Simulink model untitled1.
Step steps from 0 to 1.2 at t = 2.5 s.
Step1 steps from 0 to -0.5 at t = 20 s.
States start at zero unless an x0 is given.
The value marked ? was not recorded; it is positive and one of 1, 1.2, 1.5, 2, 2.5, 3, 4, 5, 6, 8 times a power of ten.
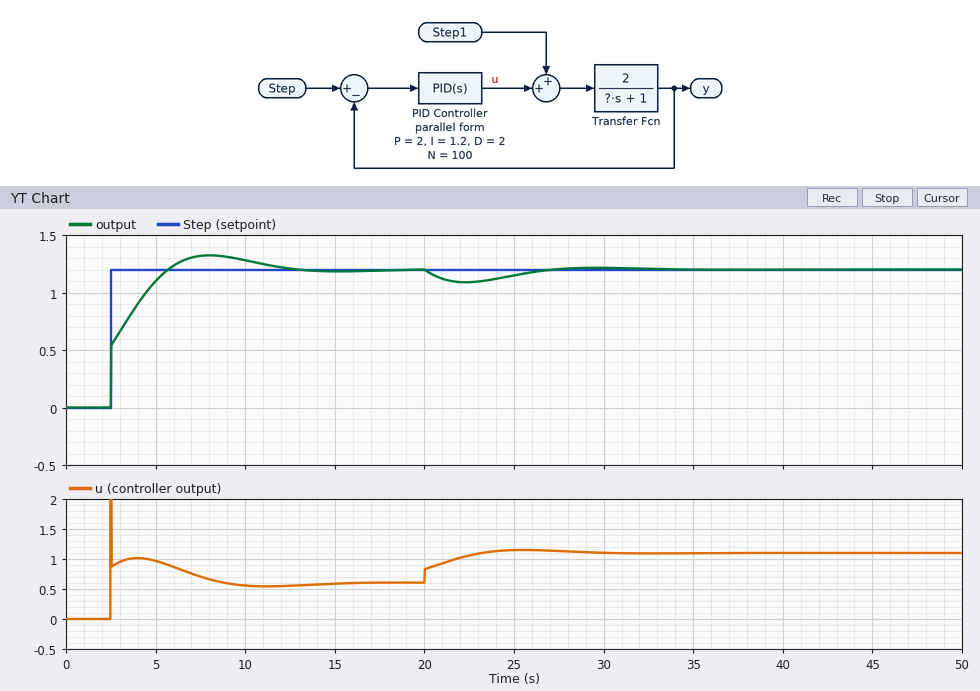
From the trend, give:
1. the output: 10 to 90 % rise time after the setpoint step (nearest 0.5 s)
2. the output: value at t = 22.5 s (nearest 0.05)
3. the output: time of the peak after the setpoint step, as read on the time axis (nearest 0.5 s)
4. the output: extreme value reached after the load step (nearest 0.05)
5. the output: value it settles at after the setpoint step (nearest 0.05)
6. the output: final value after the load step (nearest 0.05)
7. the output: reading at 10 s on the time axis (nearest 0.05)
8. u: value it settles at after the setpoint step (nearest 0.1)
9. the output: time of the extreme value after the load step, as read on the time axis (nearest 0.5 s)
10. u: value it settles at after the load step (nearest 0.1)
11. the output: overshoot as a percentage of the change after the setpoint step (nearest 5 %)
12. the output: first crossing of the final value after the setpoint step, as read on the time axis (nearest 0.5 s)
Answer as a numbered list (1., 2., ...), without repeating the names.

1. 2.5 s
2. 1.10
3. 8.0 s
4. 1.10
5. 1.20
6. 1.20
7. 1.30
8. 0.6
9. 22.5 s
10. 1.1
11. 10 %
12. 5.5 s
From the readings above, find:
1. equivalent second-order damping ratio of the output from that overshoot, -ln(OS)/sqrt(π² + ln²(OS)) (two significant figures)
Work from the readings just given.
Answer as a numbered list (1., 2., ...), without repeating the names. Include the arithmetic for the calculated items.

1. ln(0.1) = -2.303; 2.303 / sqrt(9.870 + 5.302) = 0.59
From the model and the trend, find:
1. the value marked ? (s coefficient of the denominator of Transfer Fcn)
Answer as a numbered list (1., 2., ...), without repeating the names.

1. 5
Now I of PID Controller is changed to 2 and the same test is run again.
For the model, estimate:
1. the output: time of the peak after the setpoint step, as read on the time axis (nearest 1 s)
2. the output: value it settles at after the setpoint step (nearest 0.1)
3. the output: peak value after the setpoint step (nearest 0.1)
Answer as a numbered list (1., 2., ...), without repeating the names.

1. 7 s
2. 1.2
3. 1.4
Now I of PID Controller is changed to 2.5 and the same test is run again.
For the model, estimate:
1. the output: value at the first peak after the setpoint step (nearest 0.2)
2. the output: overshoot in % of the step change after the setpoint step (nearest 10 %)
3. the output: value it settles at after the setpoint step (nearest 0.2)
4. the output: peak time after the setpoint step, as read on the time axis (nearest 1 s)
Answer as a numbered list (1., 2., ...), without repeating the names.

1. 1.4
2. 20 %
3. 1.2
4. 6 s
